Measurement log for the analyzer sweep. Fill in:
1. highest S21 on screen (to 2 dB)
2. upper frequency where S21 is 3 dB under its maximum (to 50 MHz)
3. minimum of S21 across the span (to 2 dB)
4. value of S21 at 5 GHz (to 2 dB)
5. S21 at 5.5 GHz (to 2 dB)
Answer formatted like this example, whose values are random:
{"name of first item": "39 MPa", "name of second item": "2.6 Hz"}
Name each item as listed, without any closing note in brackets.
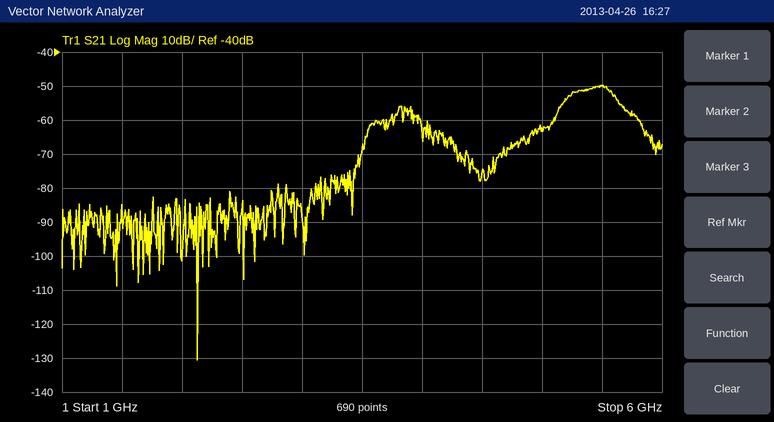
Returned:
{"highest S21 on screen": "-50 dB", "upper frequency where S21 is 3 dB under its maximum": "5.60 GHz", "minimum of S21 across the span": "-130 dB", "value of S21 at 5 GHz": "-62 dB", "S21 at 5.5 GHz": "-50 dB"}
